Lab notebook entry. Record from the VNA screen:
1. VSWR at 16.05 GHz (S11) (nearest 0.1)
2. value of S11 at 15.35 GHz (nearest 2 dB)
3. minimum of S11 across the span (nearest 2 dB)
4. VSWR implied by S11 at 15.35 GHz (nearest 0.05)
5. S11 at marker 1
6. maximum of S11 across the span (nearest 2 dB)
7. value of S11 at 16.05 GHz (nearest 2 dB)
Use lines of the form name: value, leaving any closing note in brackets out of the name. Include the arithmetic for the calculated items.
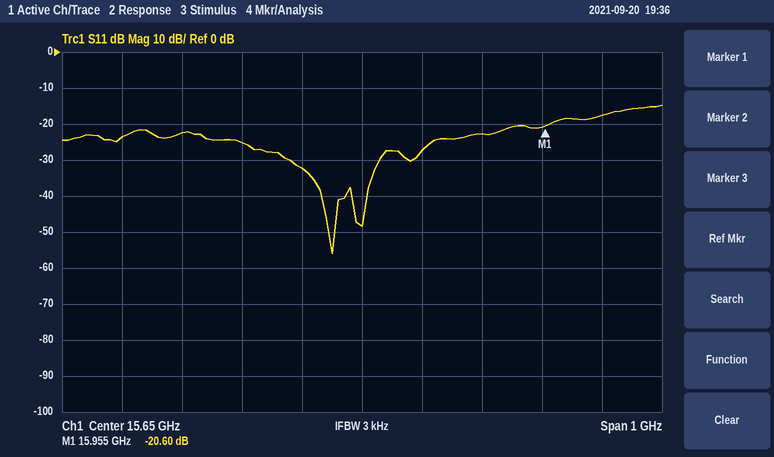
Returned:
VSWR at 16.05 GHz (S11): |Γ| = 10^(-18/20) = 0.1259; VSWR = (1 + 0.1259)/(1 − 0.1259) ≈ 1.3
value of S11 at 15.35 GHz: -22 dB
minimum of S11 across the span: -56 dB
VSWR implied by S11 at 15.35 GHz: |Γ| = 10^(-22/20) = 0.0794; VSWR = (1 + 0.0794)/(1 − 0.0794) ≈ 1.17, so 1.15 to the nearest 0.05
S11 at marker 1: -20.60 dB
maximum of S11 across the span: -14 dB
value of S11 at 16.05 GHz: -18 dB
